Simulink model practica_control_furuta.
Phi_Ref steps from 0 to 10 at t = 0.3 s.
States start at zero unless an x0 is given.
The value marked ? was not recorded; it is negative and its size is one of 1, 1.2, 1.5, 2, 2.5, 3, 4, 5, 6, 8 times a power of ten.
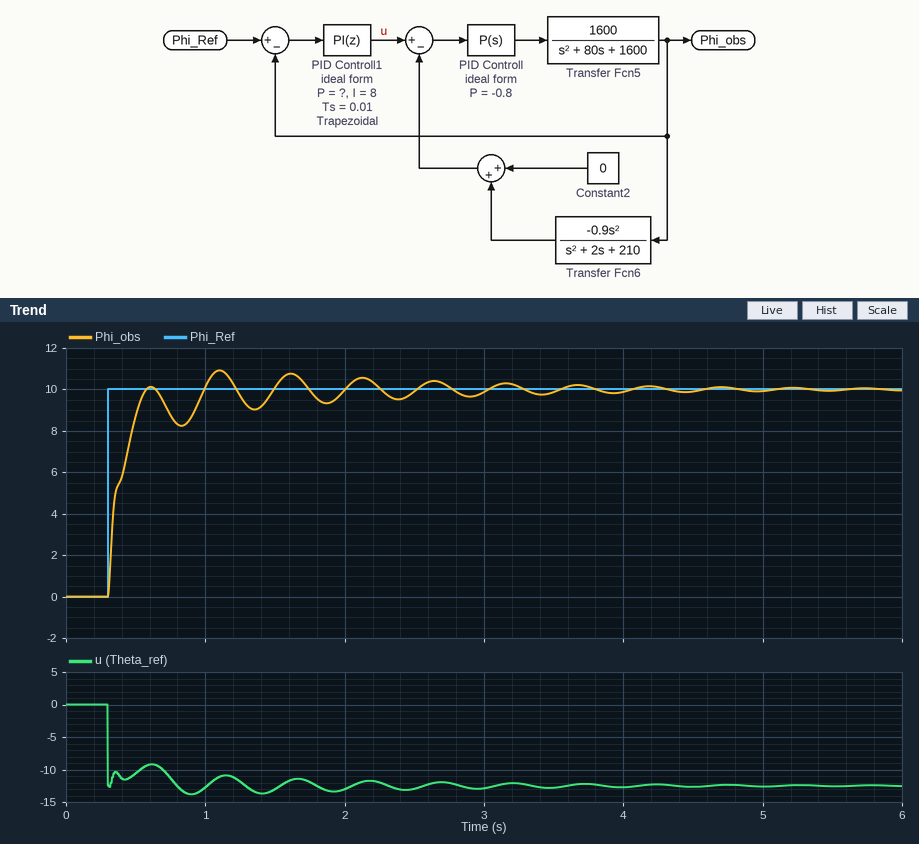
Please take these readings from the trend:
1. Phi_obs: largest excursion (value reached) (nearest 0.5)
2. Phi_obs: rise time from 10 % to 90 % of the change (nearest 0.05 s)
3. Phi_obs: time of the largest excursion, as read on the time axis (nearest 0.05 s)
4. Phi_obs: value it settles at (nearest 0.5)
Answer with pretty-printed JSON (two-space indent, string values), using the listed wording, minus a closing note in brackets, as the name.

{
  "Phi_obs: largest excursion (value reached)": "11.0",
  "Phi_obs: rise time from 10 % to 90 % of the change": "0.20 s",
  "Phi_obs: time of the largest excursion, as read on the time axis": "1.10 s",
  "Phi_obs: value it settles at": "10.0"
}
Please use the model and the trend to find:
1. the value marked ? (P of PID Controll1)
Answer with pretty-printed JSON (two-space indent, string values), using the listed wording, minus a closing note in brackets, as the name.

{
  "the value marked ?": "-1.2"
}
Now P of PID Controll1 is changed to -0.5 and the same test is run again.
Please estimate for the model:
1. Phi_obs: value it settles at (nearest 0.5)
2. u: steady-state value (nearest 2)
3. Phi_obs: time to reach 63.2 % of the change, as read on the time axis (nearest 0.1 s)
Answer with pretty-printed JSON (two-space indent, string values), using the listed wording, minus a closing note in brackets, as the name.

{
  "Phi_obs: value it settles at": "10.0",
  "u: steady-state value": "-12",
  "Phi_obs: time to reach 63.2 % of the change, as read on the time axis": "0.5 s"
}
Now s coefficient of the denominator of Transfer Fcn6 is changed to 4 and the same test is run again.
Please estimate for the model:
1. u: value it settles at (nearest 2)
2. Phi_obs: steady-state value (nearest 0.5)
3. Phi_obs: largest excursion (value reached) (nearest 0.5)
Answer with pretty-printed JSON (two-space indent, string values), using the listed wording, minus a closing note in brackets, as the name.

{
  "u: value it settles at": "-12",
  "Phi_obs: steady-state value": "10.0",
  "Phi_obs: largest excursion (value reached)": "10.5"
}
